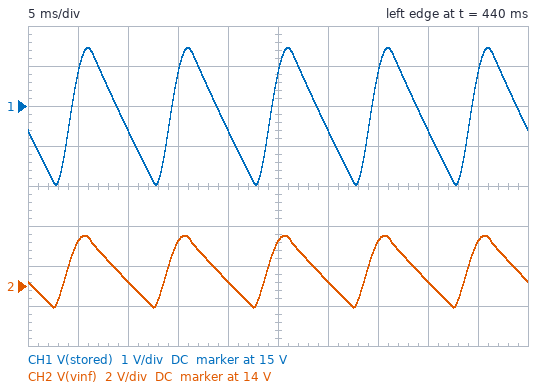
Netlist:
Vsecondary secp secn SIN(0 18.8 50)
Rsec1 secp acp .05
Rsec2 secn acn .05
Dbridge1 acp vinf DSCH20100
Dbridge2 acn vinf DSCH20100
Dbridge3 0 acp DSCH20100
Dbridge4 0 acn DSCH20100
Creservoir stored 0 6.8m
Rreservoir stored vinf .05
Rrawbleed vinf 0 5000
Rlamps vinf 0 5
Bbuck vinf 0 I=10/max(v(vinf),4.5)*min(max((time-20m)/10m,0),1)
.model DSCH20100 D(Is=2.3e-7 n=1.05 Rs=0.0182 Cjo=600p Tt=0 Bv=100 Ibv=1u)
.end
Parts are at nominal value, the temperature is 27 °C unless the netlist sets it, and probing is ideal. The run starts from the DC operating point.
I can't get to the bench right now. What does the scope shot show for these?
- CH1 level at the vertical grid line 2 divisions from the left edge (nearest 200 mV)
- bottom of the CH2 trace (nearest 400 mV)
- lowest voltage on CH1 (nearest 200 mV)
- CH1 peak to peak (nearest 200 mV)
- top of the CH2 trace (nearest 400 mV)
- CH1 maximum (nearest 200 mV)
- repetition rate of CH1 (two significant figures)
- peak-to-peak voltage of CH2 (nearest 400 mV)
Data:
14.4 V
12.8 V
13.0 V
3.4 V
16.4 V
16.4 V
100 Hz
3.6 V
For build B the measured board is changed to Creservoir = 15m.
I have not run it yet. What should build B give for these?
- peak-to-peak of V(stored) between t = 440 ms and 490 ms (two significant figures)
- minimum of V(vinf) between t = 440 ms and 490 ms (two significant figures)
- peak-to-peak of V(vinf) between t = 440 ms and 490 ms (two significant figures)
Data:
1.6 V
14 V
1.9 V
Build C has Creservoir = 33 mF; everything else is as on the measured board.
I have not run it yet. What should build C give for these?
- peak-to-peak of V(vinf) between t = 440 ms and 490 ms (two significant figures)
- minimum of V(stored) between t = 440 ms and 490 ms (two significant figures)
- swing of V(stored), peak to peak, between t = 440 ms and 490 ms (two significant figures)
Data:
1.2 V
15 V
730 mV
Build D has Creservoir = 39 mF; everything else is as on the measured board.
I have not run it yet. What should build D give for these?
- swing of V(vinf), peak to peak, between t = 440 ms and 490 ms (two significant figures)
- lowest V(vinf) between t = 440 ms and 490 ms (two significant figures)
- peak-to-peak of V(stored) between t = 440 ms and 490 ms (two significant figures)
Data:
1.1 V
15 V
620 mV
